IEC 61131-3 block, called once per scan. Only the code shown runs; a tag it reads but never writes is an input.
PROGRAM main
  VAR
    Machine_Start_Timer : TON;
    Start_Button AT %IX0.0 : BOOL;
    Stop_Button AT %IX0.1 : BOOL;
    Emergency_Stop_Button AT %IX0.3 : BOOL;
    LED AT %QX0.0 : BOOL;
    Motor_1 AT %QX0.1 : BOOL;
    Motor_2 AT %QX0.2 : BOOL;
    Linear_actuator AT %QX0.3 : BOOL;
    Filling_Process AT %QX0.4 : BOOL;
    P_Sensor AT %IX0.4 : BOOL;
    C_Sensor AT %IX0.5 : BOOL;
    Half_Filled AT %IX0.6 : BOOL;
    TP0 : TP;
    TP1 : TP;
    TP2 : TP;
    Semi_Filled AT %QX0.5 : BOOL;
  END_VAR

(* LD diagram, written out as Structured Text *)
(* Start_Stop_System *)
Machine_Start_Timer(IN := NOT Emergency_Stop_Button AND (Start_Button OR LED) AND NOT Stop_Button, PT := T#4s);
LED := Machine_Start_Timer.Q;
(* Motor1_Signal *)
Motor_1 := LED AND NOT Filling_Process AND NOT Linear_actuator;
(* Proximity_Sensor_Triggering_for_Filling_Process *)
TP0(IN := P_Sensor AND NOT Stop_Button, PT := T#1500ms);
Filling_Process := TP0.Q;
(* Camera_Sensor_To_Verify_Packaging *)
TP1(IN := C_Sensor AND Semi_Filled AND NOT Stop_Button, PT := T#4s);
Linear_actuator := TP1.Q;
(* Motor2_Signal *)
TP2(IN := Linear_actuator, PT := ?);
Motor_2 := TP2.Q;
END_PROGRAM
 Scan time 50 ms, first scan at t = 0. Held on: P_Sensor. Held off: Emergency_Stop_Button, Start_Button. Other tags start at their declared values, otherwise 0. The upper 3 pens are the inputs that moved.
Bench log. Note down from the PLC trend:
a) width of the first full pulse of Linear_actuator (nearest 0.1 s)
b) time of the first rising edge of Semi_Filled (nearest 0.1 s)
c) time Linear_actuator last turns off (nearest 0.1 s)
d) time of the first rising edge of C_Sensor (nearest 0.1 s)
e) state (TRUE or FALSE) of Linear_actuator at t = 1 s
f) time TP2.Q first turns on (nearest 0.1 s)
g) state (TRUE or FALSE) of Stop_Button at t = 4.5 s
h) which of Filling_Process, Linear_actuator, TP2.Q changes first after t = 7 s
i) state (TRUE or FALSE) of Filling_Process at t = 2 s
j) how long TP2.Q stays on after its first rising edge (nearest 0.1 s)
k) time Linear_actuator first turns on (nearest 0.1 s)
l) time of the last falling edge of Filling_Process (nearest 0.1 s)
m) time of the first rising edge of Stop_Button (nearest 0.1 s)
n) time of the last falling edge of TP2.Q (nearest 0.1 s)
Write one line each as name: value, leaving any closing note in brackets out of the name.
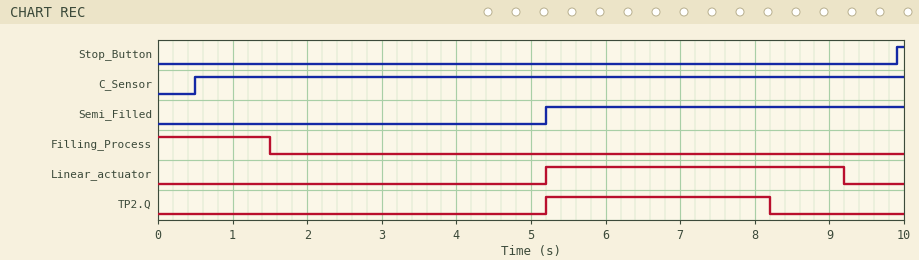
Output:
width of the first full pulse of Linear_actuator: 4.0 s
time of the first rising edge of Semi_Filled: 5.2 s
time Linear_actuator last turns off: 9.2 s
time of the first rising edge of C_Sensor: 0.5 s
state (TRUE or FALSE) of Linear_actuator at t = 1 s: FALSE
time TP2.Q first turns on: 5.2 s
state (TRUE or FALSE) of Stop_Button at t = 4.5 s: FALSE
which of Filling_Process, Linear_actuator, TP2.Q changes first after t = 7 s: TP2.Q
state (TRUE or FALSE) of Filling_Process at t = 2 s: FALSE
how long TP2.Q stays on after its first rising edge: 3.0 s
time Linear_actuator first turns on: 5.2 s
time of the last falling edge of Filling_Process: 1.5 s
time of the first rising edge of Stop_Button: 9.9 s
time of the last falling edge of TP2.Q: 8.2 s
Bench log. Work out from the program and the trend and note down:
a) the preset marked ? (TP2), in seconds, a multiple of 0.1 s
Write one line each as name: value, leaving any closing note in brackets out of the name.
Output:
the preset marked ? (TP2), in seconds, a multiple of 0.1 s: 3.0 s
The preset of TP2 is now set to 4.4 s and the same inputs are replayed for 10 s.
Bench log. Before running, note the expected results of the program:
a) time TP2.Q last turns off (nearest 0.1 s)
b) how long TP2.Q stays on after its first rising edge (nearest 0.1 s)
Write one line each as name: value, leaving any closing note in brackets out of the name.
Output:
time TP2.Q last turns off: 9.6 s
how long TP2.Q stays on after its first rising edge: 4.4 s
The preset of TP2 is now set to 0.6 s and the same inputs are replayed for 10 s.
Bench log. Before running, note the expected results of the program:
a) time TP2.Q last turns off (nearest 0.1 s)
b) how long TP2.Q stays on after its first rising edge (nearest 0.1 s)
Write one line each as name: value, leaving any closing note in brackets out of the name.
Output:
time TP2.Q last turns off: 5.8 s
how long TP2.Q stays on after its first rising edge: 0.6 s
